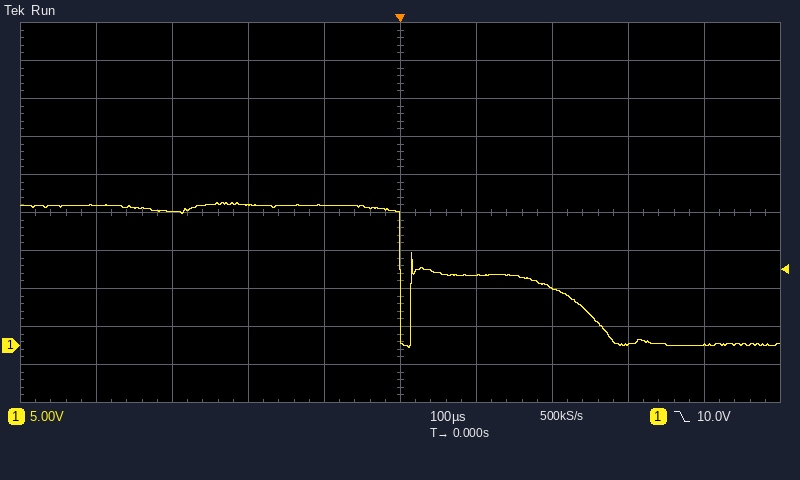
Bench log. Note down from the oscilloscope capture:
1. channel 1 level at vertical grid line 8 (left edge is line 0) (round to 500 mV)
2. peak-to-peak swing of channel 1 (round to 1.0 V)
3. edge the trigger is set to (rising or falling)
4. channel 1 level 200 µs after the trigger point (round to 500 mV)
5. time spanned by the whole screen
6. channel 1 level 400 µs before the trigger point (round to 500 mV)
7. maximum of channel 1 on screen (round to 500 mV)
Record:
0.0 V
19.0 V
falling
7.5 V
1 ms
18.5 V
19.0 V
